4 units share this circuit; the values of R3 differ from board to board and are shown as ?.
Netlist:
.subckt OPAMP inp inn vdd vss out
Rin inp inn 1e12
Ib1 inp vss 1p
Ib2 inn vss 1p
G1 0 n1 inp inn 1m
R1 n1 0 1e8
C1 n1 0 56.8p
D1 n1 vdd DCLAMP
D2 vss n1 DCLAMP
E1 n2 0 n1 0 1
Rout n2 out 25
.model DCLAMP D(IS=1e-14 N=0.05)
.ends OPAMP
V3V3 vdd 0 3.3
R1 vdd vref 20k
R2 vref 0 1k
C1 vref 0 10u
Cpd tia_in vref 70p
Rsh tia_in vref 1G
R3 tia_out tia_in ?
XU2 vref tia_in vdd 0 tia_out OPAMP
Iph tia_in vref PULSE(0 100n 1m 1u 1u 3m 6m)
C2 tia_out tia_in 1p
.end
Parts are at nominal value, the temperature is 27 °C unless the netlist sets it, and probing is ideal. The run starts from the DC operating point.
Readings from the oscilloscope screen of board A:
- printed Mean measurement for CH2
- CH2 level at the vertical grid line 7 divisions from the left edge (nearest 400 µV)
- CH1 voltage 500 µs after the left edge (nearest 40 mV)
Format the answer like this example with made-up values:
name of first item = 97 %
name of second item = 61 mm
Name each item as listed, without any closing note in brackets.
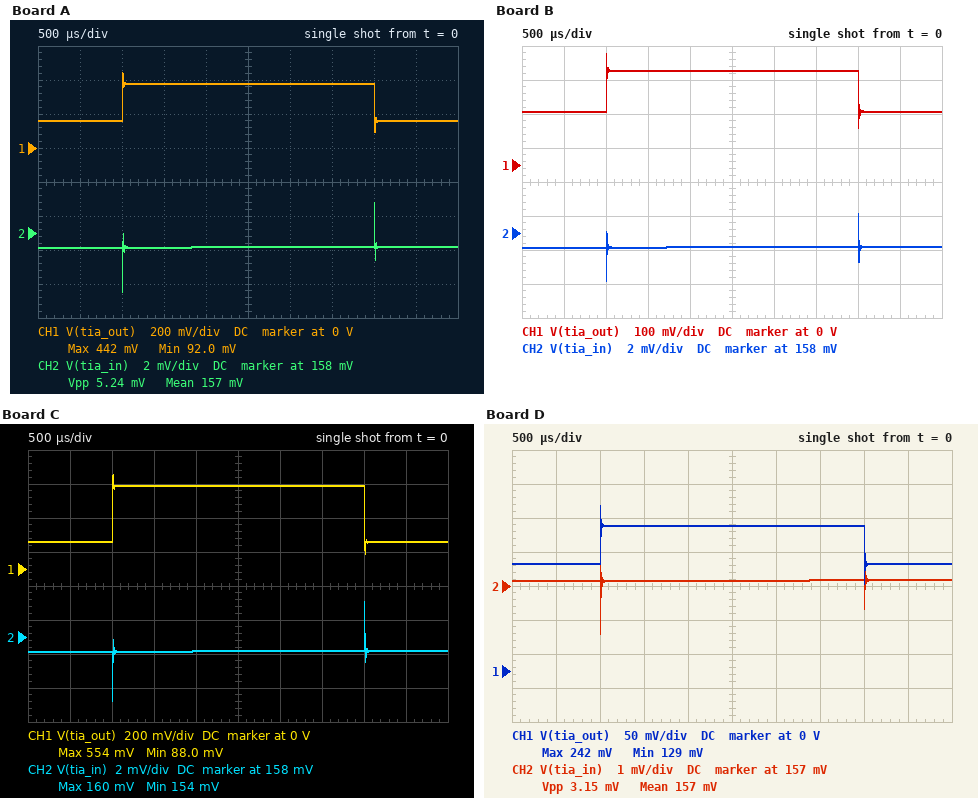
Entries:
printed Mean measurement for CH2 = 157 mV
CH2 level at the vertical grid line 7 divisions from the left edge = 157.2 mV
CH1 voltage 500 µs after the left edge = 160 mV
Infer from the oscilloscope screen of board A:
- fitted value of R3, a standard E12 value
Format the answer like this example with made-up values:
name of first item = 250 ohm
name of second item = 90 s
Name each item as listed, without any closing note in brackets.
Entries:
fitted value of R3, a standard E12 value = 2.2 MΩ
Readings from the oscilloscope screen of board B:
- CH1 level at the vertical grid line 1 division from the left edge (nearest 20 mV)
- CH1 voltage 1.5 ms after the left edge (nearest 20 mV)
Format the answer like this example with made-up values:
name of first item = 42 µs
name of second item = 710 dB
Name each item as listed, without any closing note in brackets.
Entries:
CH1 level at the vertical grid line 1 division from the left edge = 160 mV
CH1 voltage 1.5 ms after the left edge = 280 mV
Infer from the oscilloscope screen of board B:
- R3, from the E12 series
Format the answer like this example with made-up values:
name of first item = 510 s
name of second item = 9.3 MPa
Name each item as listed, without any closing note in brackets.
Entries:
R3, from the E12 series = 1.2 MΩ
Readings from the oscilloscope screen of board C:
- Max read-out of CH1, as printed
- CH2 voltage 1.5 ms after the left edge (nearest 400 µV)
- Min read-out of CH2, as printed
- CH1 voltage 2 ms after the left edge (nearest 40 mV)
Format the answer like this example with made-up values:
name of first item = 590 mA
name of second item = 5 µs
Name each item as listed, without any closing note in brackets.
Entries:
Max read-out of CH1, as printed = 554 mV
CH2 voltage 1.5 ms after the left edge = 157.2 mV
Min read-out of CH2, as printed = 154 mV
CH1 voltage 2 ms after the left edge = 480 mV
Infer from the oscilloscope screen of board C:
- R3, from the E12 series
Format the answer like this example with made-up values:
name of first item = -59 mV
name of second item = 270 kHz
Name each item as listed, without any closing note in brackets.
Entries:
R3, from the E12 series = 3.3 MΩ
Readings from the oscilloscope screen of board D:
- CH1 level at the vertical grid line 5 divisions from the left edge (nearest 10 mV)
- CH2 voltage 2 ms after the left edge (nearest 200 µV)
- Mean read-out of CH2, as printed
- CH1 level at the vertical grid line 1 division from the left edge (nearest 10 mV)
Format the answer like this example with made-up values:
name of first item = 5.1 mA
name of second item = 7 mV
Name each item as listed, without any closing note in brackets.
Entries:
CH1 level at the vertical grid line 5 divisions from the left edge = 210 mV
CH2 voltage 2 ms after the left edge = 157.2 mV
Mean read-out of CH2, as printed = 157 mV
CH1 level at the vertical grid line 1 division from the left edge = 160 mV
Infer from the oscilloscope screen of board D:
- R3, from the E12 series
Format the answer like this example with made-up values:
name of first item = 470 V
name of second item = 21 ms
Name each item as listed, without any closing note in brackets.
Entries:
R3, from the E12 series = 560 kΩ
